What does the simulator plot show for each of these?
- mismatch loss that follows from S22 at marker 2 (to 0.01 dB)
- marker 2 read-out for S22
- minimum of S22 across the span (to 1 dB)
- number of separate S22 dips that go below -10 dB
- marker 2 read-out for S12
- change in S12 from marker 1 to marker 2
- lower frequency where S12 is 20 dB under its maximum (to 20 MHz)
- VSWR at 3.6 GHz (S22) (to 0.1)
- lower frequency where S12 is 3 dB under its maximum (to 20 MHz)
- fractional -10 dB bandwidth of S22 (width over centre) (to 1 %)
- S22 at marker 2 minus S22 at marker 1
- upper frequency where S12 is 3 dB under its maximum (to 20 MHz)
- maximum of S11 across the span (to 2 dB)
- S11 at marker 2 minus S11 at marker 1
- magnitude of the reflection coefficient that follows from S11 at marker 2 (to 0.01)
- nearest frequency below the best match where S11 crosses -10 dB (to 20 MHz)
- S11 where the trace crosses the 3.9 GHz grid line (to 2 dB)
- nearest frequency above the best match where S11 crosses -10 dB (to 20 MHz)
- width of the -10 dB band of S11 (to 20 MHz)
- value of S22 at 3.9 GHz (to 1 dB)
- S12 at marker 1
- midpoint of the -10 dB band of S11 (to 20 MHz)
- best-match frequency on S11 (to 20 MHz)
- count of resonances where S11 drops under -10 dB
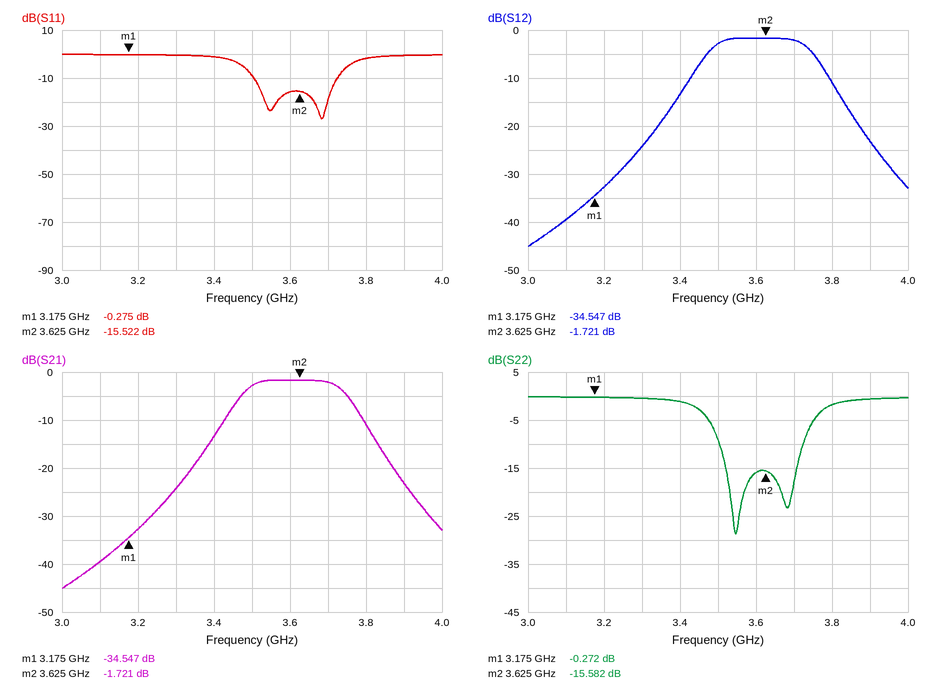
0.12 dB
-15.582 dB
-29 dB
2
-1.721 dB
32.826 dB
3.32 GHz
1.4
3.48 GHz
6 %
-15.310 dB
3.74 GHz
0 dB
-15.247 dB
0.17
3.50 GHz
0 dB
3.72 GHz
220 MHz
-1 dB
-34.547 dB
3.62 GHz
3.68 GHz
2
